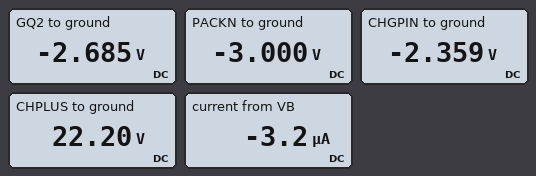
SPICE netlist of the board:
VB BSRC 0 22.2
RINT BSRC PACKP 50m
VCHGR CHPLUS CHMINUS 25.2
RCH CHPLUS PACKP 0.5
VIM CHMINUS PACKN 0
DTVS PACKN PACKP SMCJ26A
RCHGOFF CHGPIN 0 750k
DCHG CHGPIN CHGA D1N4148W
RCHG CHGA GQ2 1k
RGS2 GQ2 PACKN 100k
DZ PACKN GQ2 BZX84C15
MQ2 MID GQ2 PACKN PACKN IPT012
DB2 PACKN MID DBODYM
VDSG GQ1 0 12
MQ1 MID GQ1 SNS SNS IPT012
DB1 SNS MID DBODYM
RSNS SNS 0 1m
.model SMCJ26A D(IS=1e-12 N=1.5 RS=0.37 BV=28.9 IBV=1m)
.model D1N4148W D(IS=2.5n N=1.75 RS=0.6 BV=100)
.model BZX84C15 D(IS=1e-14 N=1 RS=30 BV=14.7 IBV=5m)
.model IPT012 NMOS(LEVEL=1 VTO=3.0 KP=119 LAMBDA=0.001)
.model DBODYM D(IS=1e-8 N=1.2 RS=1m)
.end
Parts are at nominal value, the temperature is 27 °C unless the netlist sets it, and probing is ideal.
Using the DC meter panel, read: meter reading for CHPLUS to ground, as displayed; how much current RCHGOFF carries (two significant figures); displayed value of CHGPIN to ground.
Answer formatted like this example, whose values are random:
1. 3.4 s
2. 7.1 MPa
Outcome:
1. 22.20 V
2. 3.1 µA
3. -2.359 V
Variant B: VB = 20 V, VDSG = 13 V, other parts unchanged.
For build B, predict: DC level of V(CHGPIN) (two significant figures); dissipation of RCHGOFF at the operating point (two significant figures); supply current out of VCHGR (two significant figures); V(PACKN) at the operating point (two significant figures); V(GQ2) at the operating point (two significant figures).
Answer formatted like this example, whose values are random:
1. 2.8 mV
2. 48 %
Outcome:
1. -4.3 V
2. 24 µW
3. 5.7 µA
4. -5.2 V
5. -4.6 V
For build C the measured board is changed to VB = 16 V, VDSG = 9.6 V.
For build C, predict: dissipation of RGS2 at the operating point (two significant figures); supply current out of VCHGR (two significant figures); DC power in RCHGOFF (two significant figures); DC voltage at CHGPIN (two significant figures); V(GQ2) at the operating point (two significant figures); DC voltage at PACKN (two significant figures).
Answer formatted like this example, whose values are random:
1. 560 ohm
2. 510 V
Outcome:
1. 11 µW
2. 10 µA
3. 81 µW
4. -7.8 V
5. -8.2 V
6. -9.2 V
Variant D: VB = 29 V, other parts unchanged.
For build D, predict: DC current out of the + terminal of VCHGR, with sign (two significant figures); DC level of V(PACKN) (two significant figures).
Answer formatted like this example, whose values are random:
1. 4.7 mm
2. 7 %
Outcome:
1. -5.7 A
2. 640 mV
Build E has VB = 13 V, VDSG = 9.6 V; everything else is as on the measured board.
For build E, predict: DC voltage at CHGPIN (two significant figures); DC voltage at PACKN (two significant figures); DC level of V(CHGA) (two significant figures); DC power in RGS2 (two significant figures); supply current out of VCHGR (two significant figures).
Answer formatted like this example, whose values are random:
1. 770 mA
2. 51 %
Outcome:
1. -10 V
2. -12 V
3. -11 V
4. 19 µW
5. 14 µA
